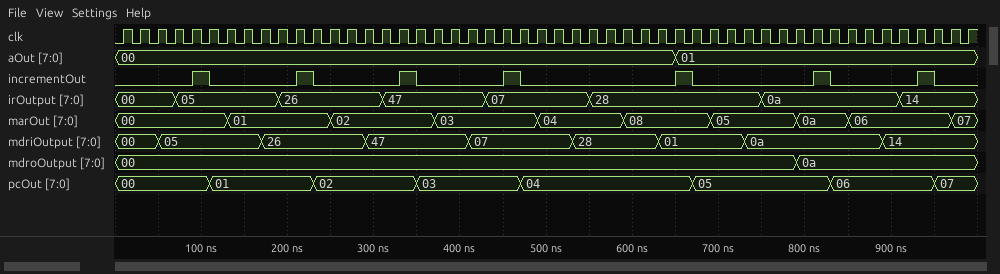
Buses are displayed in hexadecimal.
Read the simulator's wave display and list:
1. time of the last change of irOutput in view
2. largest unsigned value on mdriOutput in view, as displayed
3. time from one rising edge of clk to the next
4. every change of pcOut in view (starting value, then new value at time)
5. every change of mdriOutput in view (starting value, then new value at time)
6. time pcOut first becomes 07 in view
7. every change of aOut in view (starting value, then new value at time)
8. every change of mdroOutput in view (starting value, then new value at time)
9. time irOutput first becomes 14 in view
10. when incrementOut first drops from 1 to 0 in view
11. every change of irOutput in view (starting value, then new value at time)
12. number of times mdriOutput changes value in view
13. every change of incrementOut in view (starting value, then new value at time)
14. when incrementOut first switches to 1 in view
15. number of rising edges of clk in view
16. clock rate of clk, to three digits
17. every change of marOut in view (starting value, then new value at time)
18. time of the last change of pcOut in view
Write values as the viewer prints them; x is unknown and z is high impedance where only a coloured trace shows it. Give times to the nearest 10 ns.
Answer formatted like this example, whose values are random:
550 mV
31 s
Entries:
910 ns
47
20 ns
00, 01 at 110 ns, 02 at 230 ns, 03 at 350 ns, 04 at 470 ns, 05 at 670 ns, 06 at 830 ns, 07 at 950 ns
00, 05 at 50 ns, 26 at 170 ns, 47 at 290 ns, 07 at 410 ns, 28 at 530 ns, 01 at 630 ns, 0a at 730 ns, 14 at 890 ns
950 ns
00, 01 at 650 ns
00, 0a at 790 ns
910 ns
110 ns
00, 05 at 70 ns, 26 at 190 ns, 47 at 310 ns, 07 at 430 ns, 28 at 550 ns, 0a at 750 ns, 14 at 910 ns
8
0, 1 at 90 ns, 0 at 110 ns, 1 at 210 ns, 0 at 230 ns, 1 at 330 ns, 0 at 350 ns, 1 at 450 ns, 0 at 470 ns, 1 at 650 ns, 0 at 670 ns, 1 at 810 ns, 0 at 830 ns, 1 at 930 ns, 0 at 950 ns
90 ns
50
50.0 MHz
00, 01 at 130 ns, 02 at 250 ns, 03 at 370 ns, 04 at 490 ns, 08 at 590 ns, 05 at 690 ns, 0a at 790 ns, 06 at 850 ns, 07 at 970 ns
950 ns
